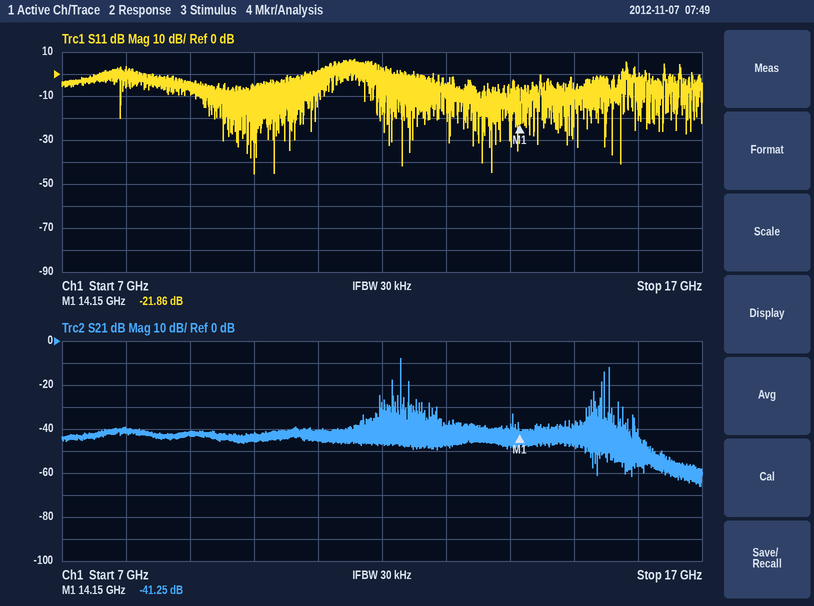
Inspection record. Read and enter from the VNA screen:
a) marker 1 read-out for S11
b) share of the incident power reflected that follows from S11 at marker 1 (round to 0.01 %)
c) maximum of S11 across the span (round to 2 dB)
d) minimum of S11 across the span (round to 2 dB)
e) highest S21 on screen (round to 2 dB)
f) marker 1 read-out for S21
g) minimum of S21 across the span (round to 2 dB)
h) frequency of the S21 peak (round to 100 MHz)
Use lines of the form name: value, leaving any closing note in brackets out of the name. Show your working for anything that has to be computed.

marker 1 read-out for S11: -21.86 dB
share of the incident power reflected that follows from S11 at marker 1: 10^(-21.86/10) ≈ 0.65 %
maximum of S11 across the span: 6 dB
minimum of S11 across the span: -46 dB
highest S21 on screen: -8 dB
marker 1 read-out for S21: -41.25 dB
minimum of S21 across the span: -66 dB
frequency of the S21 peak: 12.3 GHz
